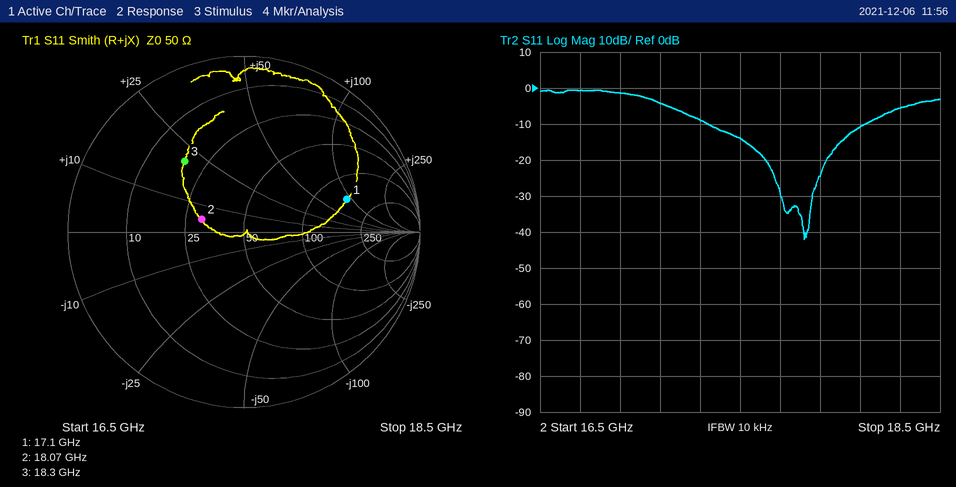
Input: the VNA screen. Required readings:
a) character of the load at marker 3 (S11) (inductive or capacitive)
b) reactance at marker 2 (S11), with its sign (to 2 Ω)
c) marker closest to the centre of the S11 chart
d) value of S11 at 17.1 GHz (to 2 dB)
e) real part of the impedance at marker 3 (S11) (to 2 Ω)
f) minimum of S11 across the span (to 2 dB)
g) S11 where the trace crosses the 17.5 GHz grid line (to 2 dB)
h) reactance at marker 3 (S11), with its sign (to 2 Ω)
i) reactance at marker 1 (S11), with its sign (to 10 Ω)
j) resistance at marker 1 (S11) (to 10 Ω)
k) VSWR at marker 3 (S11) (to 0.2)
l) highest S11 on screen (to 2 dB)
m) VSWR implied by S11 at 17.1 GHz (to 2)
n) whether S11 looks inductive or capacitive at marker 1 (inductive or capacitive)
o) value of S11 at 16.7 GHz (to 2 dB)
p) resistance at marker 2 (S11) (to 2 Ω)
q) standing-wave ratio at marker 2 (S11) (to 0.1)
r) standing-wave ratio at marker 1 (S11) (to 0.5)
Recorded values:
inductive
+4 Ω
marker 2
-4 dB
18 Ω
-42 dB
-14 dB
+20 Ω
+90 Ω
150 Ω
3.2
0 dB
4
inductive
0 dB
30 Ω
1.7
4.0
